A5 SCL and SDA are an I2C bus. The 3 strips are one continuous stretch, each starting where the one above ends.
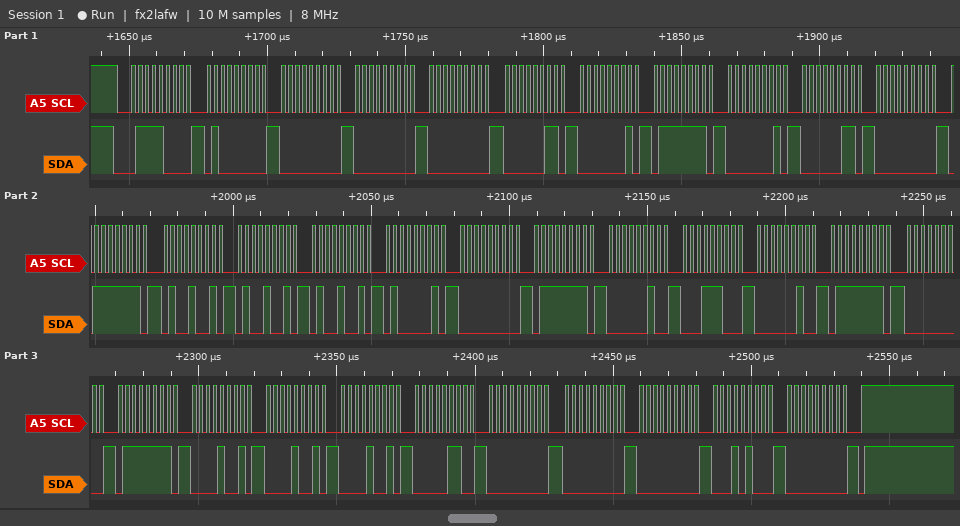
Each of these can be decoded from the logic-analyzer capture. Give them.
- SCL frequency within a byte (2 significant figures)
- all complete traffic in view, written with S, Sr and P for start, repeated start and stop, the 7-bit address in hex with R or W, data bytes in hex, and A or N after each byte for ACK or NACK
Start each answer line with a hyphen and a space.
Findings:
- 400 kHz
- S 3CW A 40 A 00 A 00 A 00 A 03 A 01 A 7F A 01 A 03 A 00 A 7F A 49 A 49 A 49 A 41 A 00 A 7F A 02 A 1C A 02 A 7F A 00 A 7F A 09 A 09 A 09 A 06 A 00 A 00 A 00 A 14 A 00 A P
